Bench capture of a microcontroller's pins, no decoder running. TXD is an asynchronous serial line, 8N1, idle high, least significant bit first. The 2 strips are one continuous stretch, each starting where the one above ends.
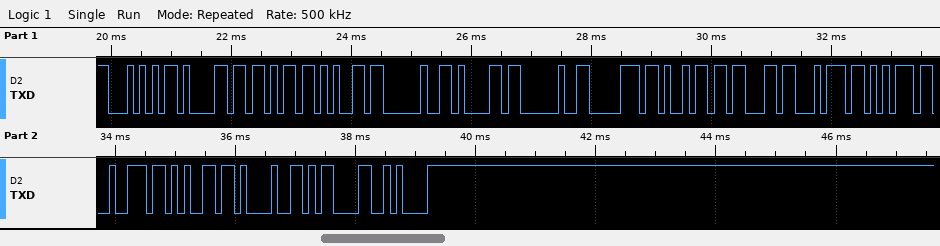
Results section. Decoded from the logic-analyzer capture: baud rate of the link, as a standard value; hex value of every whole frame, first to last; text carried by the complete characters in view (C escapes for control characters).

9600 baud
0x54 0x61 0x6B 0x65 0x20 0x61 0x20 0x70 0x69 0x63 0x74 0x75 0x72 0x65 0x21 0x0D 0x0A
"Take a picture!\r\n"
